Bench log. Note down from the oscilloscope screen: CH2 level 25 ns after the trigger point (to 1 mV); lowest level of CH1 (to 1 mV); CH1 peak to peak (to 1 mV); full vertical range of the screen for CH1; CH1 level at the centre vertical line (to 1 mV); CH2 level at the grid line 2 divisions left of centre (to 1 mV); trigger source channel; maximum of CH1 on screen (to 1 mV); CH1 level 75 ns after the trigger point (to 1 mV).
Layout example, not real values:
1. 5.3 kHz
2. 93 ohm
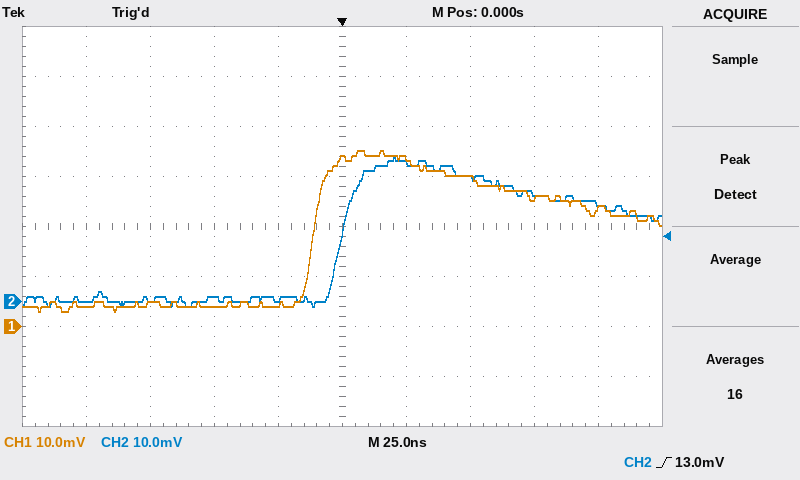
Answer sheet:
1. 28 mV
2. 3 mV
3. 32 mV
4. 80 mV
5. 34 mV
6. 1 mV
7. CH2
8. 35 mV
9. 26 mV
